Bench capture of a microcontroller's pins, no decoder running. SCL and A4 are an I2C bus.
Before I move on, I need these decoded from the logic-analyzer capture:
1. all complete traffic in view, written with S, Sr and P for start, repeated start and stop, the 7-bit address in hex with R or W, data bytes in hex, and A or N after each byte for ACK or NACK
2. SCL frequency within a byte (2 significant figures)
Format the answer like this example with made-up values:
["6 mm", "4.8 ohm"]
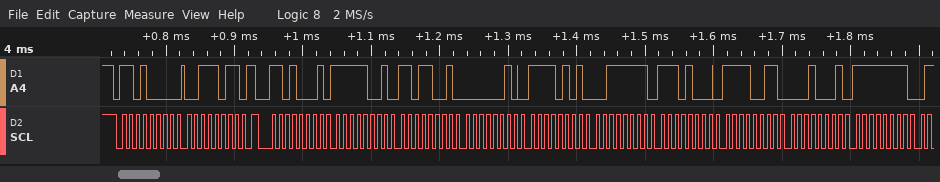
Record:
["S 68W A 3B A Sr 68R A F9 A D9 A 02 A F5 A 3F A E8 A F3 A 11 A FF A", "100 kHz"]
